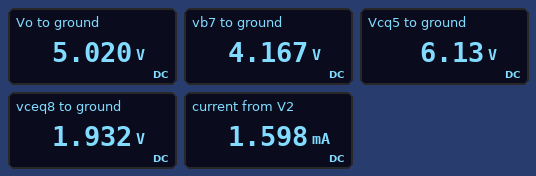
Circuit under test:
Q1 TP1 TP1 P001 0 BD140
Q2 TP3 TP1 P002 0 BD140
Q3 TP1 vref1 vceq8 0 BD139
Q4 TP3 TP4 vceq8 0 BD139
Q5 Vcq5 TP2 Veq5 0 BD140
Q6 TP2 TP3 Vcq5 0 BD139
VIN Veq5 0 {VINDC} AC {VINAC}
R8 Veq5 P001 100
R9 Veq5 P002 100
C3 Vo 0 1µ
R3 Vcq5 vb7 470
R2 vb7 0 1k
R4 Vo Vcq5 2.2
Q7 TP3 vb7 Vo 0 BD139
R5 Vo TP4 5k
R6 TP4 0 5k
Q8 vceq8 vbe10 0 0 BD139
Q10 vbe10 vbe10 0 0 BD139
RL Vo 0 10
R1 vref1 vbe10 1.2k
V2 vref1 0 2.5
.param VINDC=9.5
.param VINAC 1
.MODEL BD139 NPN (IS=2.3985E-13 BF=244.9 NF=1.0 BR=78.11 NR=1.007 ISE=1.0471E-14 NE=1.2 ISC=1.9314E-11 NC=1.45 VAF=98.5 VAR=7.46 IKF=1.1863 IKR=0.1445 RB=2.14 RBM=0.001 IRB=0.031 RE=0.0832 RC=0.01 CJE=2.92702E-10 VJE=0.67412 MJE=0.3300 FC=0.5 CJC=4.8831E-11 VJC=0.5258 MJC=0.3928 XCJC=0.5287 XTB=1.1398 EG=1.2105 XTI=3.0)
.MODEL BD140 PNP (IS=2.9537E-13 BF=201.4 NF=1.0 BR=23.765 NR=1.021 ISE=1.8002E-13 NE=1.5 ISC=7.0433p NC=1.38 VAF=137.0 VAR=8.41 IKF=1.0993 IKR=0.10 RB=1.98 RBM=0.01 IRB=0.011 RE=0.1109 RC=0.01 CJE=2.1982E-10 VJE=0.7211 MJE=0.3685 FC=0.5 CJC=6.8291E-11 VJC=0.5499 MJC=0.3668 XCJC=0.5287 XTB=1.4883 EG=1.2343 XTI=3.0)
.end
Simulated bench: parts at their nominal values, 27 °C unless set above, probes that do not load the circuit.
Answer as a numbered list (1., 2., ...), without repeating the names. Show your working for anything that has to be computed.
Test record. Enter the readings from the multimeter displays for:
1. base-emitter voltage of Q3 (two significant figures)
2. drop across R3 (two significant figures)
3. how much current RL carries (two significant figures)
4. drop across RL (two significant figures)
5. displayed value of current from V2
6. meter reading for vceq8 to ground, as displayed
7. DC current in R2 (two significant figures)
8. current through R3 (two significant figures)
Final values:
1. 2.5 V - 1.932 V = 570 mV
2. 6.13 V - 4.167 V = 2.0 V
3. (5.02 V) / 10 Ω = 500 mA
4. 5.02 V = 5.0 V
5. 1.598 mA
6. 1.932 V
7. (4.167 V) / 1 kΩ = 4.2 mA
8. (6.13 V - 4.167 V) / 470 Ω = 4.2 mA
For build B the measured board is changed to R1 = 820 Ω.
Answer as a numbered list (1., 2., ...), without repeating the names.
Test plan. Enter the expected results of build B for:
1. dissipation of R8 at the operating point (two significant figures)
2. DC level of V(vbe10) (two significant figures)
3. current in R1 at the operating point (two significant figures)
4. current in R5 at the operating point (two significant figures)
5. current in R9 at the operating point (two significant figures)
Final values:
1. 140 µW
2. 600 mV
3. 2.3 mA
4. 510 µA
5. 1.2 mA
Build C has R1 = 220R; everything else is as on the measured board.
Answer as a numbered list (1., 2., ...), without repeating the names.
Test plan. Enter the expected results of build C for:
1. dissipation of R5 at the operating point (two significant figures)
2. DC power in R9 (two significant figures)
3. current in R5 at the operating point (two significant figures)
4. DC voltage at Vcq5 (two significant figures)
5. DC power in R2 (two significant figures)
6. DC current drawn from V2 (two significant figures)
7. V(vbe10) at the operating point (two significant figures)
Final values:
1. 1.4 mW
2. 1.8 mW
3. 520 µA
4. 6.2 V
5. 18 mW
6. 8.5 mA
7. 630 mV
